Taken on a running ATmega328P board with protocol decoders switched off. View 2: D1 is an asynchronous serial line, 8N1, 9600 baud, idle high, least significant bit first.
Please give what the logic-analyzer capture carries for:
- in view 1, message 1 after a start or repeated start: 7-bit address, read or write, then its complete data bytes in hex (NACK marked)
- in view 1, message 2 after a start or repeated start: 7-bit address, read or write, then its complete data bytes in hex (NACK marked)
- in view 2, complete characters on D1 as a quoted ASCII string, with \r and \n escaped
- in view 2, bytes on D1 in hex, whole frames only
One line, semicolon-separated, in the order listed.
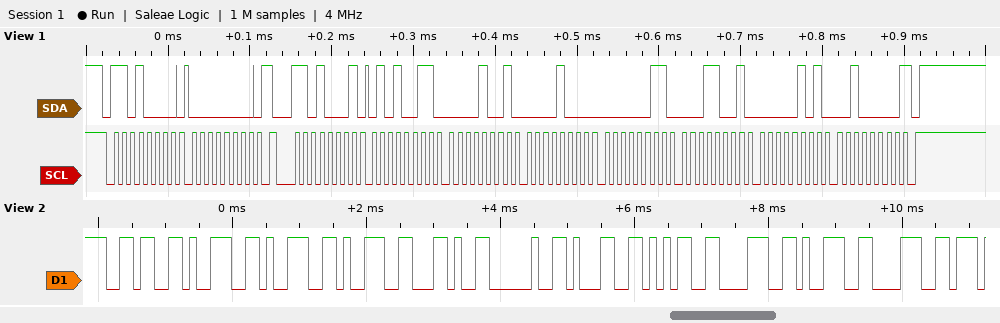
0x68 write: 00; 0x68 read: 53 09 08 03 19 05 20 NACK; "6999, 15898"; 36 39 39 39 2C 20 31 35 38 39 38
